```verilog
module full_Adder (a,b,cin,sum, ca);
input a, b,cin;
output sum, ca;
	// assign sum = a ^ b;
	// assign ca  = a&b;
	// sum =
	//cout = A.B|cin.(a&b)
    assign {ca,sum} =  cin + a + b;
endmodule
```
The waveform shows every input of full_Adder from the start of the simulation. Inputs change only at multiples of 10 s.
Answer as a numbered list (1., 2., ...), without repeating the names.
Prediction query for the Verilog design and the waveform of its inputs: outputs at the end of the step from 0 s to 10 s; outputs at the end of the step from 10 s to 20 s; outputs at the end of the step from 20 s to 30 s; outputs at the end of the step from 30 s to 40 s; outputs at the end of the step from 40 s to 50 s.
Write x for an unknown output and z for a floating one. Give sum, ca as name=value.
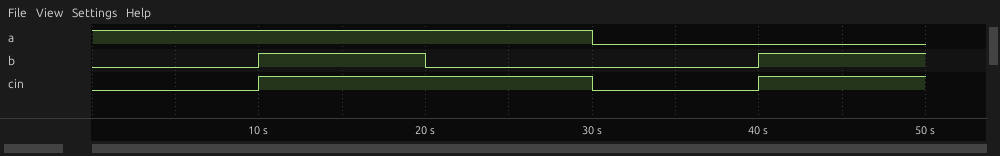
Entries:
1. sum=1, ca=0
2. sum=1, ca=1
3. sum=0, ca=1
4. sum=0, ca=0
5. sum=0, ca=1
